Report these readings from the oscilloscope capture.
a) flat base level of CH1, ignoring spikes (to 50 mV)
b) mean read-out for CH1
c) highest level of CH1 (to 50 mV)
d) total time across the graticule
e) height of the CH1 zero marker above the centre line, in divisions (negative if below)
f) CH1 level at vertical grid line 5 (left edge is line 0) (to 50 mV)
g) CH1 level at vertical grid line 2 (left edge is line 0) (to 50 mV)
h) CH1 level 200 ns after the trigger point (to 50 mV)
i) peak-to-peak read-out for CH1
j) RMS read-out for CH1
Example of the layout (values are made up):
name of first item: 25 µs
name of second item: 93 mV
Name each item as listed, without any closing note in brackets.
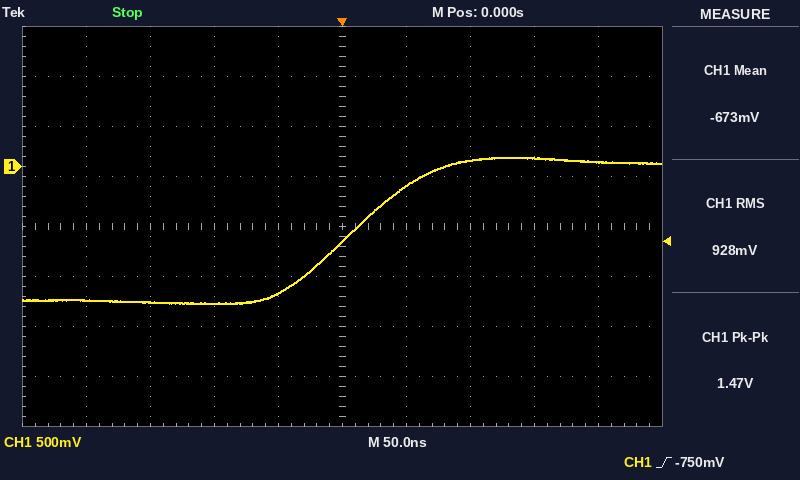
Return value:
flat base level of CH1, ignoring spikes: -1.35 V
mean read-out for CH1: -673 mV
highest level of CH1: 100 mV
total time across the graticule: 500 ns
height of the CH1 zero marker above the centre line, in divisions: +1.2 div
CH1 level at vertical grid line 5 (left edge is line 0): -750 mV
CH1 level at vertical grid line 2 (left edge is line 0): -1.35 V
CH1 level 200 ns after the trigger point: 50 mV
peak-to-peak read-out for CH1: 1.47 V
RMS read-out for CH1: 928 mV
